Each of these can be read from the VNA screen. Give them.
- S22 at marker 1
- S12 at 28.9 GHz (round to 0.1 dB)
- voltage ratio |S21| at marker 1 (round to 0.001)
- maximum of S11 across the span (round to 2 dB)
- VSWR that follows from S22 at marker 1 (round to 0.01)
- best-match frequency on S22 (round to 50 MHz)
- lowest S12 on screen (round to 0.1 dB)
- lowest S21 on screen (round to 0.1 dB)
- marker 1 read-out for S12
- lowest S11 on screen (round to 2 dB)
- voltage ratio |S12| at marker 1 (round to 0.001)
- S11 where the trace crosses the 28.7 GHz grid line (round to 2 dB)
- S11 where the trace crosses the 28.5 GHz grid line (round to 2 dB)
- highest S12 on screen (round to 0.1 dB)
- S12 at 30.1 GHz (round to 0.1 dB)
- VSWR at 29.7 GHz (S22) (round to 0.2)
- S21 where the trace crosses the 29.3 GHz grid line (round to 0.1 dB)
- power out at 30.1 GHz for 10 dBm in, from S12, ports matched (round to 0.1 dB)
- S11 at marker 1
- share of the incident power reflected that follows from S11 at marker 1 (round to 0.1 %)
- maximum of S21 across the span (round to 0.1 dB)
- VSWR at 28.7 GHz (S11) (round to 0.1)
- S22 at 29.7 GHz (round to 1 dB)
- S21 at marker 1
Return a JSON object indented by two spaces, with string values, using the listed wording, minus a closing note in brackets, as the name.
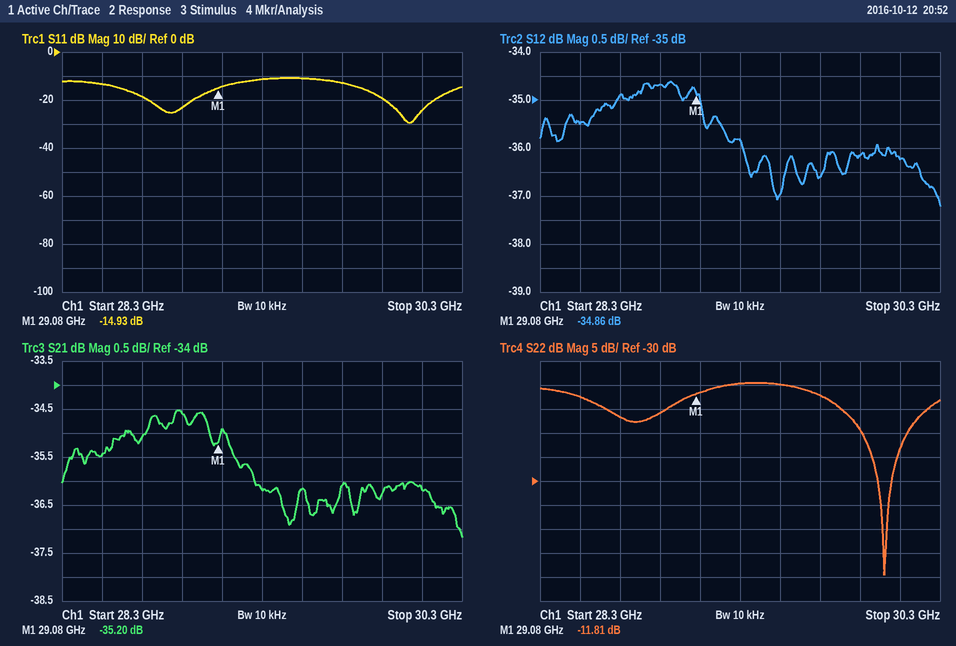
{
  "S22 at marker 1": "-11.81 dB",
  "S12 at 28.9 GHz": "-34.7 dB",
  "voltage ratio |S21| at marker 1": "0.017",
  "maximum of S11 across the span": "-10 dB",
  "VSWR that follows from S22 at marker 1": "1.69",
  "best-match frequency on S22": "30.00 GHz",
  "lowest S12 on screen": "-37.2 dB",
  "lowest S21 on screen": "-37.2 dB",
  "marker 1 read-out for S12": "-34.86 dB",
  "lowest S11 on screen": "-30 dB",
  "voltage ratio |S12| at marker 1": "0.018",
  "S11 where the trace crosses the 28.7 GHz grid line": "-18 dB",
  "S11 where the trace crosses the 28.5 GHz grid line": "-14 dB",
  "highest S12 on screen": "-34.6 dB",
  "S12 at 30.1 GHz": "-36.2 dB",
  "VSWR at 29.7 GHz (S22)": "1.6",
  "S21 where the trace crosses the 29.3 GHz grid line": "-36.2 dB",
  "power out at 30.1 GHz for 10 dBm in, from S12, ports matched": "-26.2 dBm",
  "S11 at marker 1": "-14.93 dB",
  "share of the incident power reflected that follows from S11 at marker 1": "3.2 %",
  "maximum of S21 across the span": "-34.5 dB",
  "VSWR at 28.7 GHz (S11)": "1.3",
  "S22 at 29.7 GHz": "-12 dB",
  "S21 at marker 1": "-35.20 dB"
}
